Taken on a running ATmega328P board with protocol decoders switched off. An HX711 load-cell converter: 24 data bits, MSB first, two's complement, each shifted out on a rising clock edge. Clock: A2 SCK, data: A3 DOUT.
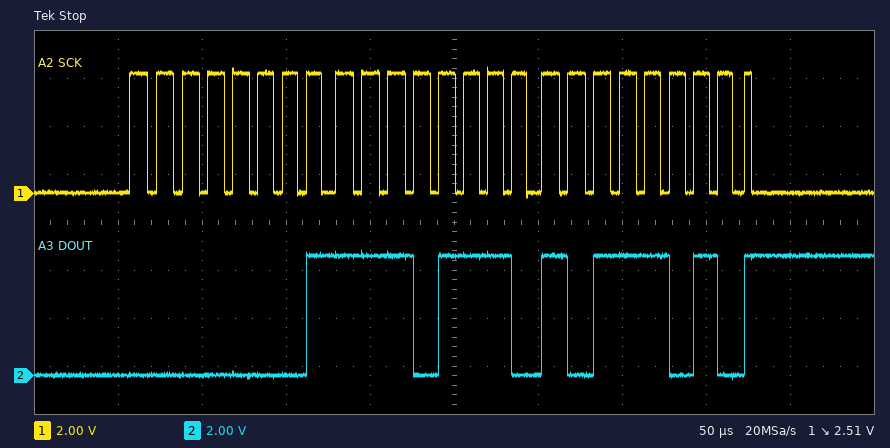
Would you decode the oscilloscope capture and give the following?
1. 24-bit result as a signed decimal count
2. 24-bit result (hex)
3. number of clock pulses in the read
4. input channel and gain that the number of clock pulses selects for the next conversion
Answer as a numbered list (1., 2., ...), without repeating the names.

1. 126650
2. 0x01EEBA
3. 25
4. channel A, gain 128
